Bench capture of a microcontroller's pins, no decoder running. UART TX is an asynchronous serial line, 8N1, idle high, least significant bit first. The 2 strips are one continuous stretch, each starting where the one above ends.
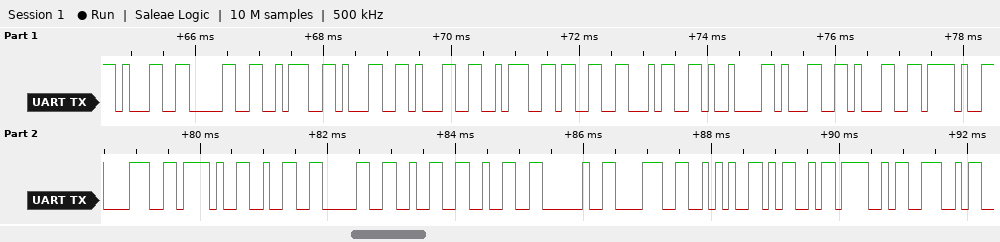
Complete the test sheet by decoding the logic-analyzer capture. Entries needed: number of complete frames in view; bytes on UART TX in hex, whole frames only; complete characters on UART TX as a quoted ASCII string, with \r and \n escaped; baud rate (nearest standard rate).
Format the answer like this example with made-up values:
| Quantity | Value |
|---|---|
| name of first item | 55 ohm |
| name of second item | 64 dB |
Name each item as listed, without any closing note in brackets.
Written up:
| Quantity | Value |
|---|---|
| number of complete frames in view | 24 |
| bytes on UART TX in hex, whole frames only | 31 30 3A 31 31 3A 33 34 09 31 31 2F 38 2F 32 30 32 32 20 38 2A 4D 4F 4E |
| complete characters on UART TX as a quoted ASCII string, with \r and \n escaped | "10:11:34\t11/8/2022 8*MON" |
| baud rate | 9600 baud |
